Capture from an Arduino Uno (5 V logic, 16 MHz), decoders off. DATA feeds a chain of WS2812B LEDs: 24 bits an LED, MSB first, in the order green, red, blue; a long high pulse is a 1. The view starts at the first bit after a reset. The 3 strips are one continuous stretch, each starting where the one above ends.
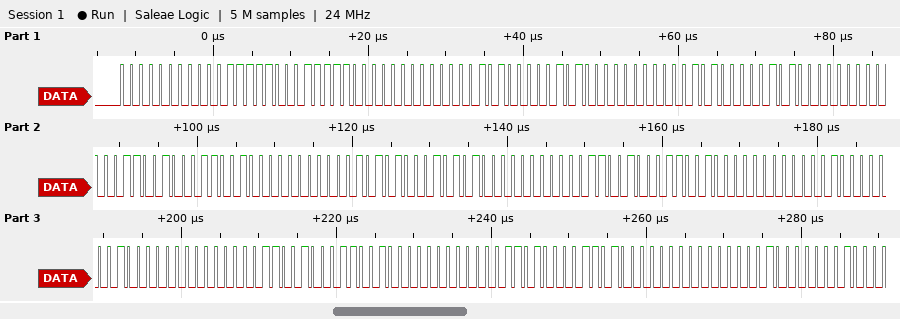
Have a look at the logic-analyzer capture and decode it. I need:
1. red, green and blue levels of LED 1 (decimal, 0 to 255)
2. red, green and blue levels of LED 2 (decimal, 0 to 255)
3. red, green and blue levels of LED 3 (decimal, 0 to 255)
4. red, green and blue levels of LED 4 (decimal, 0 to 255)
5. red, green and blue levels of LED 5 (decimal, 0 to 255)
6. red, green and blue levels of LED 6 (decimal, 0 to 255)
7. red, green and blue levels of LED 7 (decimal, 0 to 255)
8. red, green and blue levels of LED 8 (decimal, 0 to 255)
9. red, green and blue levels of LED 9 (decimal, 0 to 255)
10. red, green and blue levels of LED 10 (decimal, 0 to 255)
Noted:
31, 0, 31
5, 0, 5
20, 0, 20
50, 0, 50
42, 0, 42
50, 0, 50
16, 0, 16
50, 0, 50
26, 0, 26
2, 0, 2
